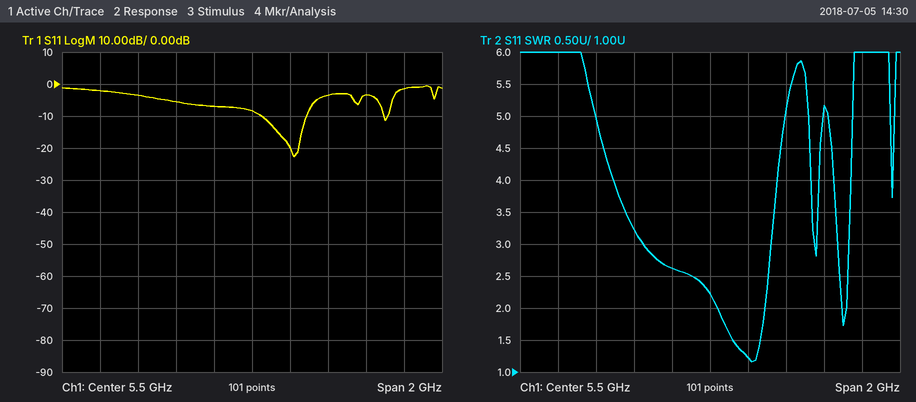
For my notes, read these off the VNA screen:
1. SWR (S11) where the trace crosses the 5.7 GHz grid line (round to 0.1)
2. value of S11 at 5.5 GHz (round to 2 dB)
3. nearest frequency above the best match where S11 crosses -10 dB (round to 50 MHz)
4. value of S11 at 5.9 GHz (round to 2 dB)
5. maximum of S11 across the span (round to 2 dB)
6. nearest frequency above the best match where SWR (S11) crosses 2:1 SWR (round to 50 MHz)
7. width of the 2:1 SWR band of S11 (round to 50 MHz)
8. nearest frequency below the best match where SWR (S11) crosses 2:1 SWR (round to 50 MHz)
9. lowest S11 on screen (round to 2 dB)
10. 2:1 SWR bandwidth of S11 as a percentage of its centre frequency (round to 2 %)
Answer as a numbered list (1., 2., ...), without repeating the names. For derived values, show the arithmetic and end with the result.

1. 1.2
2. -8 dB
3. 5.80 GHz
4. -4 dB
5. 0 dB
6. 5.80 GHz
7. 5.80 GHz − 5.55 GHz = 250 MHz
8. 5.55 GHz
9. -22 dB
10. 250 MHz / 5.675 GHz ≈ 4 %
